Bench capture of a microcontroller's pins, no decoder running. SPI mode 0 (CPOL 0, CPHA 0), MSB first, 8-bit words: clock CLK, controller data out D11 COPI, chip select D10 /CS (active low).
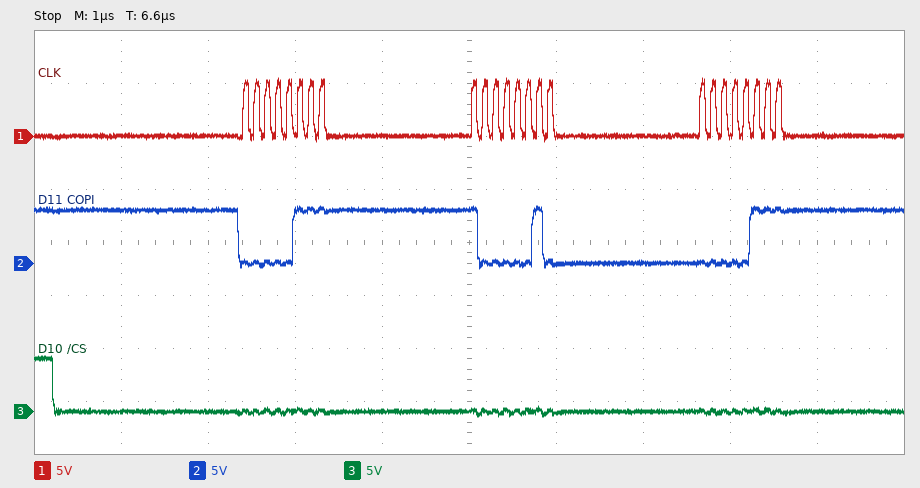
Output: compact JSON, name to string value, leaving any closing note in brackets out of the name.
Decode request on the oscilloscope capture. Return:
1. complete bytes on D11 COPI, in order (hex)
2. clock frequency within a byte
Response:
{"complete bytes on D11 COPI, in order": "0x07 0x82 0x07", "clock frequency within a byte": "8 MHz"}
